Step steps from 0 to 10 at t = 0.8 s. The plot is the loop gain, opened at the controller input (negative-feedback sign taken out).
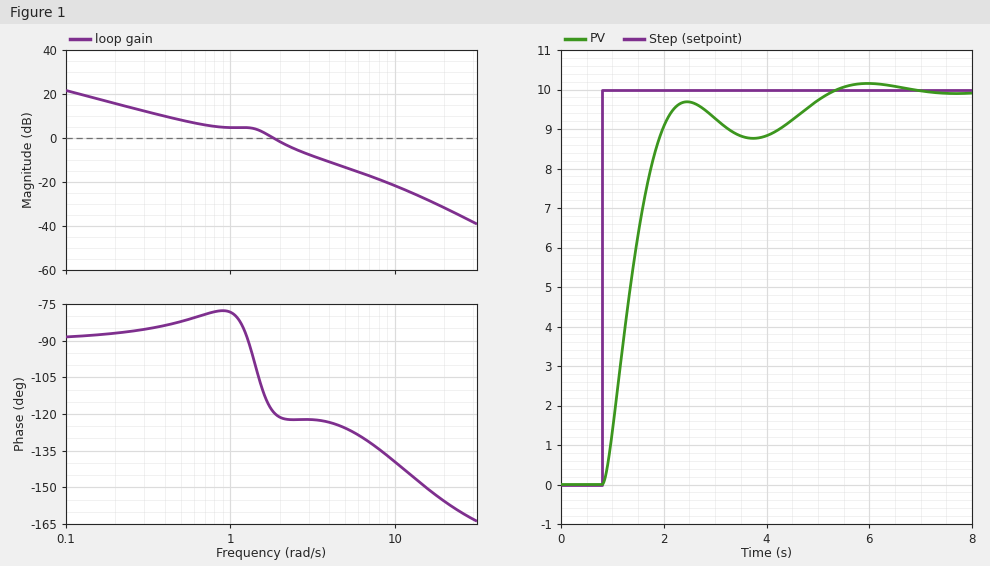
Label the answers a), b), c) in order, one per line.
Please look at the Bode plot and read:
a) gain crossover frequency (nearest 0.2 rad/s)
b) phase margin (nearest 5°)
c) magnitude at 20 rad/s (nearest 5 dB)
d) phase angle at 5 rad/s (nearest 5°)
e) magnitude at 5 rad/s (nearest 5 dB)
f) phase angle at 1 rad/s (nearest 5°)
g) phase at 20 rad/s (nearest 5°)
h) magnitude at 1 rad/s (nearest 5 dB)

a) 1.8 rad/s
b) 60°
c) -30 dB
d) -125°
e) -15 dB
f) -80°
g) -155°
h) 5 dB
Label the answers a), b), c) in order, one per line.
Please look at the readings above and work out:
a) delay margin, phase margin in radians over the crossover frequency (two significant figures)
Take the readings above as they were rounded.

a) 0.58 s
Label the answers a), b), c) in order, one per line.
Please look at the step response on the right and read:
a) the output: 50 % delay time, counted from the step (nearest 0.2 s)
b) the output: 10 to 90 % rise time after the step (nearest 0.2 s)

a) 0.6 s
b) 1.0 s
